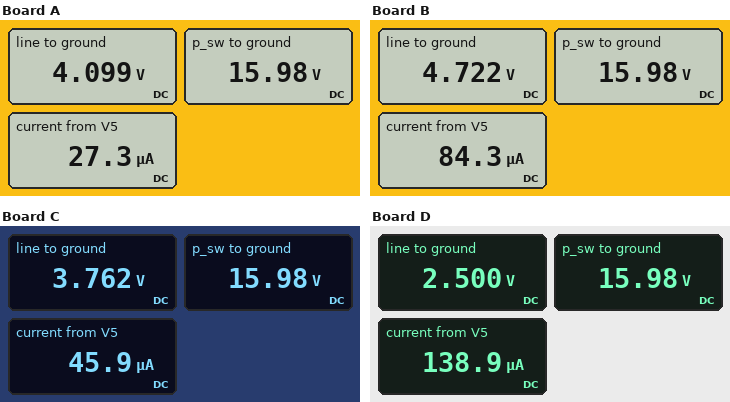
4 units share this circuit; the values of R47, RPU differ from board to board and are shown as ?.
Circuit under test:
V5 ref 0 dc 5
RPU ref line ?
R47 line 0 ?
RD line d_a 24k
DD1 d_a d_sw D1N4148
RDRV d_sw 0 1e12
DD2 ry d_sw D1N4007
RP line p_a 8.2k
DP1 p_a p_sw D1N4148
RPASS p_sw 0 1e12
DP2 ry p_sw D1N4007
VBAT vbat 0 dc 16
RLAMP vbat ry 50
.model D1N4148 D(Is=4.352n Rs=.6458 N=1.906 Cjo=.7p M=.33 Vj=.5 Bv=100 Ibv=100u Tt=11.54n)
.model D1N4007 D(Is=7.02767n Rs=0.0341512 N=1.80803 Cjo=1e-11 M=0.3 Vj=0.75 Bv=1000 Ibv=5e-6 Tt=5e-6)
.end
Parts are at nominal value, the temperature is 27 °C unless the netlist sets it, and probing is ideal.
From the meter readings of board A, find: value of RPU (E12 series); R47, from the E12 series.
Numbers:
33 kΩ
150 kΩ
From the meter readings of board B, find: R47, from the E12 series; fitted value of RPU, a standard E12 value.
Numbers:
56 kΩ
3.3 kΩ
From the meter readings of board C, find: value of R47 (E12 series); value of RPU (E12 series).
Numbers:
82 kΩ
27 kΩ
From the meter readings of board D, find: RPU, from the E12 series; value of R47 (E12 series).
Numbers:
18 kΩ
18 kΩ
